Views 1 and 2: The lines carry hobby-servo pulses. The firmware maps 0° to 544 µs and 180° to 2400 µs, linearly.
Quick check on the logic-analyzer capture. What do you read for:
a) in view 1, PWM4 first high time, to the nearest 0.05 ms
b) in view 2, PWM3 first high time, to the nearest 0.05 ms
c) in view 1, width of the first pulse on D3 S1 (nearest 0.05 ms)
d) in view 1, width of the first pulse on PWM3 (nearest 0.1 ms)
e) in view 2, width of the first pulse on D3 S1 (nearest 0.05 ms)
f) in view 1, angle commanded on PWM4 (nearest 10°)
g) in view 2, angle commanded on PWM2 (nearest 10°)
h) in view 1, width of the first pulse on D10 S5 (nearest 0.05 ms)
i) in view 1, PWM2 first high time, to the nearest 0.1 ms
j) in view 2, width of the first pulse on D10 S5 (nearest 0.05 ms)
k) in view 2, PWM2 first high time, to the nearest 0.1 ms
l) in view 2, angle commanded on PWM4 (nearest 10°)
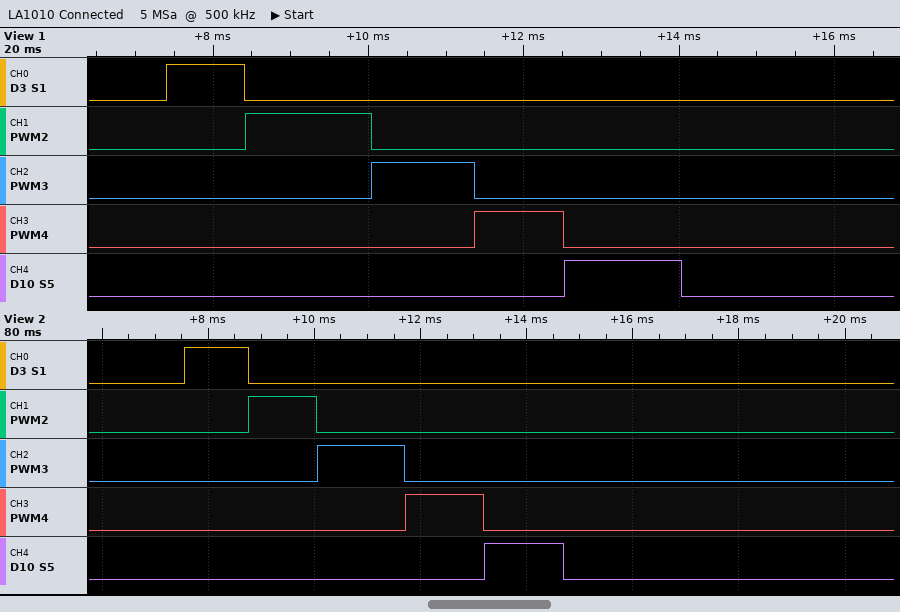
1.15 ms
1.65 ms
1.00 ms
1.3 ms
1.20 ms
60°
70°
1.50 ms
1.6 ms
1.50 ms
1.3 ms
90°
